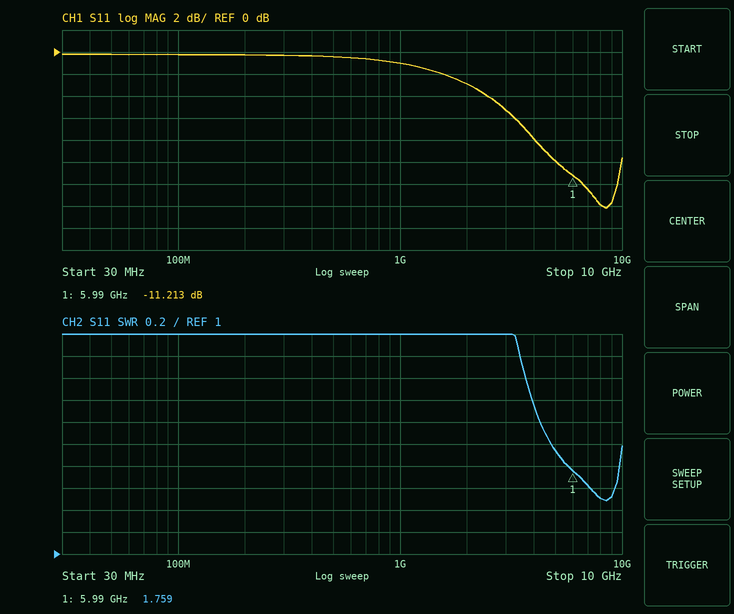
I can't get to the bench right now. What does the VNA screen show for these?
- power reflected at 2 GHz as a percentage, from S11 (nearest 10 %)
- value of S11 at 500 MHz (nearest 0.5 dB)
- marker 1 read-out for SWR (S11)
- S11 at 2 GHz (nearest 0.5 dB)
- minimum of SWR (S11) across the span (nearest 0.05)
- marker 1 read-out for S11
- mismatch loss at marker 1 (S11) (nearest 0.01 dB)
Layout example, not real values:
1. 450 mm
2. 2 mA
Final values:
1. 50 %
2. -0.5 dB
3. 1.759
4. -3.0 dB
5. 1.50
6. -11.213 dB
7. 0.34 dB
